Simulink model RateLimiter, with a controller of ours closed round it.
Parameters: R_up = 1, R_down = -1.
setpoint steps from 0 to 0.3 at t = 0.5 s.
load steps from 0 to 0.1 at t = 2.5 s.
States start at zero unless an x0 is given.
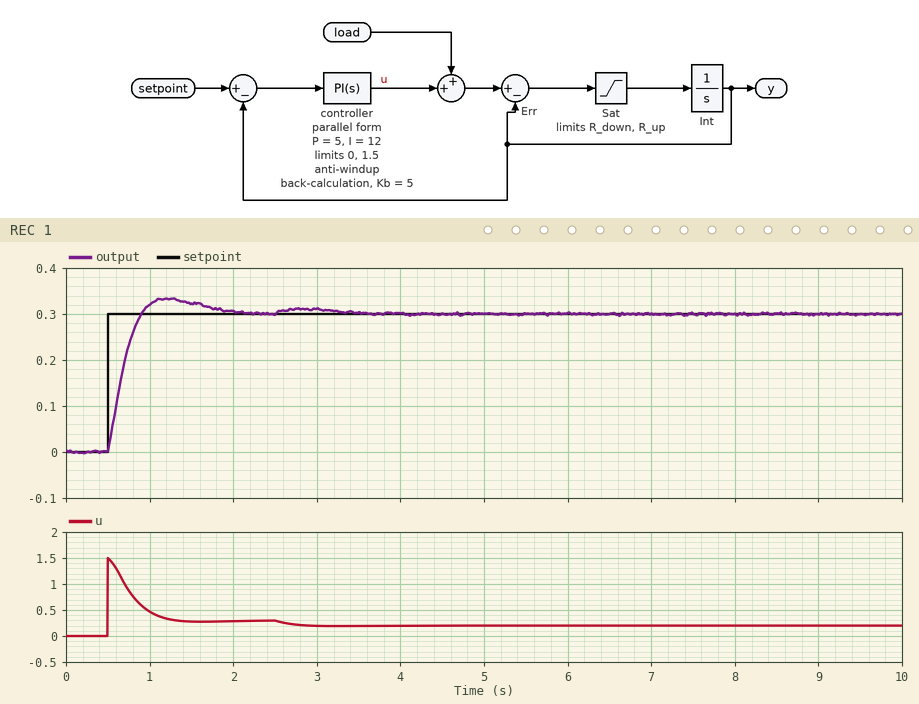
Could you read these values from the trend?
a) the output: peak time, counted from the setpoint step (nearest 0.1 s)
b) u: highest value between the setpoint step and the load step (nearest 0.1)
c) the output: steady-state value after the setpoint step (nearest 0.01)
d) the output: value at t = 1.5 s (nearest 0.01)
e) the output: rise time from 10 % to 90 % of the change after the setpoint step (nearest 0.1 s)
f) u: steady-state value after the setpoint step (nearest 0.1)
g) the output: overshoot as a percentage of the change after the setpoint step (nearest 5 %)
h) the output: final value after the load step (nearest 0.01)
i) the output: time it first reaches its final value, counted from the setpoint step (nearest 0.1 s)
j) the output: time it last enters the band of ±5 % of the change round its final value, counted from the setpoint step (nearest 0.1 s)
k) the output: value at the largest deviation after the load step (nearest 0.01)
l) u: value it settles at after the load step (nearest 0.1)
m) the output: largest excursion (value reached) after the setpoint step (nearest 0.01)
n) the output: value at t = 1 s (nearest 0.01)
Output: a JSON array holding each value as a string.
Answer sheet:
["0.7 s", "1.5", "0.30", "0.32", "0.3 s", "0.3", "10 %", "0.30", "0.4 s", "1.2 s", "0.31", "0.2", "0.33", "0.32"]
